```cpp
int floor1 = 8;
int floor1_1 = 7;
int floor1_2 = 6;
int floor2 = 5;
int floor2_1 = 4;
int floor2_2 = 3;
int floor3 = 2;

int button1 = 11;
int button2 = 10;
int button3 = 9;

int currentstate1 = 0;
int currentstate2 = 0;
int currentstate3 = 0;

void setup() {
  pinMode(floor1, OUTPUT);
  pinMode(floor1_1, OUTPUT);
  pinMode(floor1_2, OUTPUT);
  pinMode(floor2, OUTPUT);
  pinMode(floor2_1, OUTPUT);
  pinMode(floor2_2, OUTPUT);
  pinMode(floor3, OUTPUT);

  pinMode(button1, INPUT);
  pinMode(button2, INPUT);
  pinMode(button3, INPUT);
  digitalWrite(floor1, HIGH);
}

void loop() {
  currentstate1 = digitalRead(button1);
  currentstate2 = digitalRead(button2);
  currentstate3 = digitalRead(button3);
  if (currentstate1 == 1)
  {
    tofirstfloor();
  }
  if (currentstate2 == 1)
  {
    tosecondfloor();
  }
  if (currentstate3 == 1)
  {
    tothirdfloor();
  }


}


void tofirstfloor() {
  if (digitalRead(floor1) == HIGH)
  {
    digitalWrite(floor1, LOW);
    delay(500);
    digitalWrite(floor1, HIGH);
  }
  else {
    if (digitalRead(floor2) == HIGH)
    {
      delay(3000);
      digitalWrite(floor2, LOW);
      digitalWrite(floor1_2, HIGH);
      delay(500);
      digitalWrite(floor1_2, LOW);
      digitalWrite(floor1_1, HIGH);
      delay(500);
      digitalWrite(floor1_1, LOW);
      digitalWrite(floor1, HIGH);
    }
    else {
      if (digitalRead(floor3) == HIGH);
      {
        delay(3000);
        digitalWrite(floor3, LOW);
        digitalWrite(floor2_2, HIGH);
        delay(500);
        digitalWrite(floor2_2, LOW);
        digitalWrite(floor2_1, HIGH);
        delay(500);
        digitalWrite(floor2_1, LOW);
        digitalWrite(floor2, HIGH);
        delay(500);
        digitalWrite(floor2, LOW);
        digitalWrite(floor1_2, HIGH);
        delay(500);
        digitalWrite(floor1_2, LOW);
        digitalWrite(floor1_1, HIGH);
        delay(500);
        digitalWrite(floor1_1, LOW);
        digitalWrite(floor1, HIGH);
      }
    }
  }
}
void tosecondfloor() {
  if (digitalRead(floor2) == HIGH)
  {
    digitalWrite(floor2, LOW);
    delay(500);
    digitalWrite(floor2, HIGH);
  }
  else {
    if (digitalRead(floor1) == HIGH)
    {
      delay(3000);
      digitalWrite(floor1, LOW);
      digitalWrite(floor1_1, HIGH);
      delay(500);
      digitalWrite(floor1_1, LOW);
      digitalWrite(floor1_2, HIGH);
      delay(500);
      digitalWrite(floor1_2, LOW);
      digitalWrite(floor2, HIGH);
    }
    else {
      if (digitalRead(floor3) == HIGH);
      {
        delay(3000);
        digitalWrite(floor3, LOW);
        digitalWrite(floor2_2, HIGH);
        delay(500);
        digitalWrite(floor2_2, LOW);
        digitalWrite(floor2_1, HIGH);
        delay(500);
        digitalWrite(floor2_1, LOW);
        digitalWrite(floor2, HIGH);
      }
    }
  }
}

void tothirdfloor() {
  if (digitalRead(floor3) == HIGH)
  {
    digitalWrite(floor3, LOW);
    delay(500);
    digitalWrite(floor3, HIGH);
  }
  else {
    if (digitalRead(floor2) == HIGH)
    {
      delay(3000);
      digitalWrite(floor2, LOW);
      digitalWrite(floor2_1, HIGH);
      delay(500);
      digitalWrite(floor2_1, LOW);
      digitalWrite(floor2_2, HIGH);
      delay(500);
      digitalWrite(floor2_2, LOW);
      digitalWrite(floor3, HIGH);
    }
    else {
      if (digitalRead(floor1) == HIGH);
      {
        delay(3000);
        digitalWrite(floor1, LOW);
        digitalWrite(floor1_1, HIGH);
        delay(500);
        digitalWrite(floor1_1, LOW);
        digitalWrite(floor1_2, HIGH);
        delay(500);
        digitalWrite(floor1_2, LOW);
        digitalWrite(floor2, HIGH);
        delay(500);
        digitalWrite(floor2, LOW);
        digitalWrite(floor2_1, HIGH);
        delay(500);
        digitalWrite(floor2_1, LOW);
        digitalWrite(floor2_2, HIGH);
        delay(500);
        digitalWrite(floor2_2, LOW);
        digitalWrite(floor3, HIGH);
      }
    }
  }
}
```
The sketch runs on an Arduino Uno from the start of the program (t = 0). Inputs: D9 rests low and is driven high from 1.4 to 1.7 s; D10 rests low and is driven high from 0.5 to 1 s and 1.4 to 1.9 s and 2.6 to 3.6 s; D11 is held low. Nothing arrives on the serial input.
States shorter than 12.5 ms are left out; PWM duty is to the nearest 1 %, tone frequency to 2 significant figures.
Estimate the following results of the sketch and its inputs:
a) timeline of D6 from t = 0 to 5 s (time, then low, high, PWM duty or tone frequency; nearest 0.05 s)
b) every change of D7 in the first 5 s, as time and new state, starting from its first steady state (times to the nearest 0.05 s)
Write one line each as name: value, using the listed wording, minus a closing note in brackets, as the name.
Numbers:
timeline of D6 from t = 0 to 5 s: 0 s low; 4 s high; 4.5 s low
every change of D7 in the first 5 s, as time and new state, starting from its first steady state: 0 s low; 3.5 s high; 4 s low
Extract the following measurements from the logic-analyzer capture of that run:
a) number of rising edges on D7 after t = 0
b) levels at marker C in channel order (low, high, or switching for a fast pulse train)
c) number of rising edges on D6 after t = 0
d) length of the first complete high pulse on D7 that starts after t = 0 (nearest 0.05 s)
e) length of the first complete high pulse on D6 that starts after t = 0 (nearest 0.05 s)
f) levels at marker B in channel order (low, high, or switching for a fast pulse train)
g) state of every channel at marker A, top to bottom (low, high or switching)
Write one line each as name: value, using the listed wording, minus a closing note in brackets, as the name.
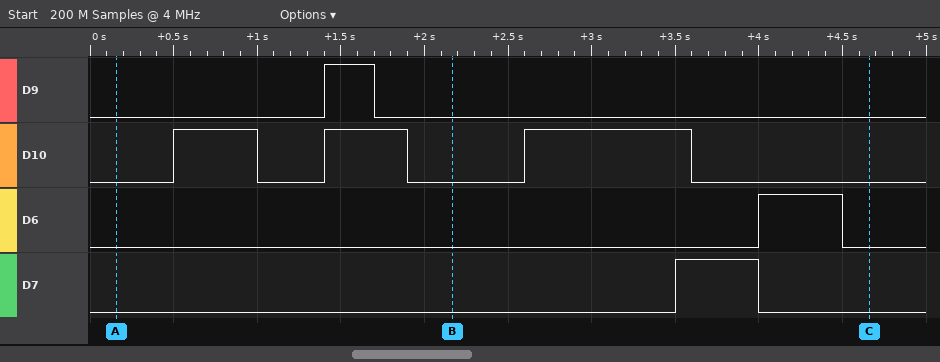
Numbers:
number of rising edges on D7 after t = 0: 1
levels at marker C in channel order: D9 low, D10 low, D6 low, D7 low
number of rising edges on D6 after t = 0: 1
length of the first complete high pulse on D7 that starts after t = 0: 0.50 s
length of the first complete high pulse on D6 that starts after t = 0: 0.50 s
levels at marker B in channel order: D9 low, D10 low, D6 low, D7 low
state of every channel at marker A, top to bottom: D9 low, D10 low, D6 low, D7 low
